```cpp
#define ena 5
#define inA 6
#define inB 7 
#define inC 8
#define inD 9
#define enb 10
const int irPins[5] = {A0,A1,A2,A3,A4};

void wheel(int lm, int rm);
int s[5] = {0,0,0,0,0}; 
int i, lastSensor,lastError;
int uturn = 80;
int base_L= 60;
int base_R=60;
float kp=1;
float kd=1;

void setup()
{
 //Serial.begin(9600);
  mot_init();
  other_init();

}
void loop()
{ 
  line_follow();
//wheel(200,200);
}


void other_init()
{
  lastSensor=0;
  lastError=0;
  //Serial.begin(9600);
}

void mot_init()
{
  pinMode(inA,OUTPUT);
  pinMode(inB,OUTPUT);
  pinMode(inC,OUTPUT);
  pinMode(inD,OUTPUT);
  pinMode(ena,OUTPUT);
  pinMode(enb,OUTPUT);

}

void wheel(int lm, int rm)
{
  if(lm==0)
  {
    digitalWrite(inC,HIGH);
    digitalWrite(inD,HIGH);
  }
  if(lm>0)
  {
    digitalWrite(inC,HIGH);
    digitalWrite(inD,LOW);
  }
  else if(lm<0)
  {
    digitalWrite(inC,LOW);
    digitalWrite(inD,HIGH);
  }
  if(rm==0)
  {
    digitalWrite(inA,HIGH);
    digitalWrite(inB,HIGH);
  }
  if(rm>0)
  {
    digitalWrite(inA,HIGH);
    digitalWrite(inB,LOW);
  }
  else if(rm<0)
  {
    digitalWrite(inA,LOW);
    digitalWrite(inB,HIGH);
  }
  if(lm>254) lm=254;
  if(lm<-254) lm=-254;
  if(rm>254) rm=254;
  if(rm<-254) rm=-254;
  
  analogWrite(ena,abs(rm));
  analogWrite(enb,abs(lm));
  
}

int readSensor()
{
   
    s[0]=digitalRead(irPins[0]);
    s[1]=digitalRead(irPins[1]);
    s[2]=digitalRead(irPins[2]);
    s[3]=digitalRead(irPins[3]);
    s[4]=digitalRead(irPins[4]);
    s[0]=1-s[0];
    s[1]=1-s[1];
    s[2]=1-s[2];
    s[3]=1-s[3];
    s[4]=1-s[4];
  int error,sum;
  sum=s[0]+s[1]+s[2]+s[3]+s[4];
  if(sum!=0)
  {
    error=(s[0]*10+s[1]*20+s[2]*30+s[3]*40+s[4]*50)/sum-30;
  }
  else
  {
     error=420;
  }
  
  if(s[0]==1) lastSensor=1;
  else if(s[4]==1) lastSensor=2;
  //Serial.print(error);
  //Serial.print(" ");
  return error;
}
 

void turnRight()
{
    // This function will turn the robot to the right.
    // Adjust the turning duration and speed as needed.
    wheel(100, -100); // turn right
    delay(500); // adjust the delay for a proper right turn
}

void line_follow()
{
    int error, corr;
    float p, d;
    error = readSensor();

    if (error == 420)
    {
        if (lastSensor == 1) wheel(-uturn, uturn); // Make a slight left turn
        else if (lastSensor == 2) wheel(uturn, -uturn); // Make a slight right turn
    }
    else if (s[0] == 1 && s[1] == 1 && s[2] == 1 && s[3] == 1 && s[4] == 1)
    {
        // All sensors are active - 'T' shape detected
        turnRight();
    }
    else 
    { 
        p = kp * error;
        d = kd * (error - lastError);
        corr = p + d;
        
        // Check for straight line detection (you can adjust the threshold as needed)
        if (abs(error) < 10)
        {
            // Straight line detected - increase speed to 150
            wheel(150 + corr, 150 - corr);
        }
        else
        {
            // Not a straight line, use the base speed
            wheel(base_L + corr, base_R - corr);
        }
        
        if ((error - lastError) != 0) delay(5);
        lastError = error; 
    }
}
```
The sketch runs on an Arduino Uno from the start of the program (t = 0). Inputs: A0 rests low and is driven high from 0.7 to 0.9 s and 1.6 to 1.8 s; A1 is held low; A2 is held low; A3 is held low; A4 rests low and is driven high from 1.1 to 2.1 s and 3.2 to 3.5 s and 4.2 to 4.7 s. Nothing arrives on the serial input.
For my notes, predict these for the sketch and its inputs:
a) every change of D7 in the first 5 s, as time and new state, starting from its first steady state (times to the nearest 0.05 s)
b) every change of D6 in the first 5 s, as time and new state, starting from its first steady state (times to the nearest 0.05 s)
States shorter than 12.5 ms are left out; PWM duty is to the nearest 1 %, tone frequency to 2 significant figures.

0 s high; 1.5 s low; 2.1 s high; 4.6 s low; 4.7 s high
0 s low; 1.5 s high; 2.1 s low; 4.6 s high; 4.7 s low
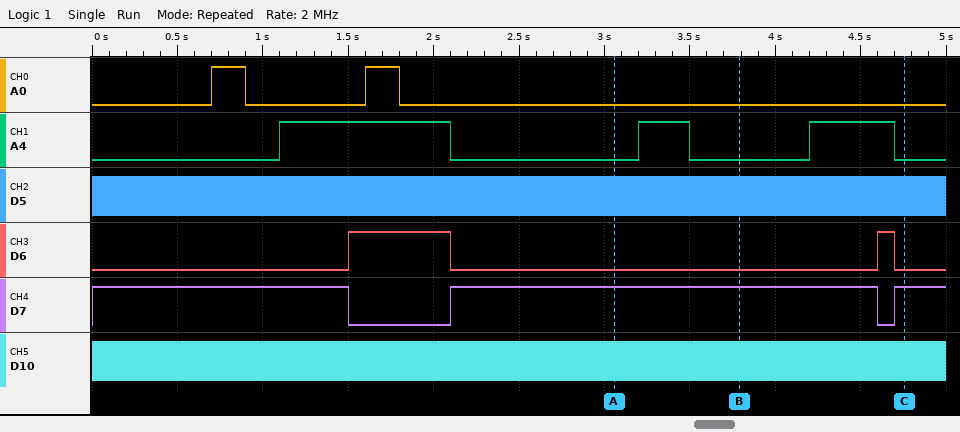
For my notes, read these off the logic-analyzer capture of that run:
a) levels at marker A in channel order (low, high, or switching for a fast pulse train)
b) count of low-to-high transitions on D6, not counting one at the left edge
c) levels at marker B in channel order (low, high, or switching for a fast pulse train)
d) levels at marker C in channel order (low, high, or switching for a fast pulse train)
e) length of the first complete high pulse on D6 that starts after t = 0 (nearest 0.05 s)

A0 low, A4 low, D5 switching, D6 low, D7 high, D10 switching
2
A0 low, A4 low, D5 switching, D6 low, D7 high, D10 switching
A0 low, A4 low, D5 switching, D6 low, D7 high, D10 switching
0.60 s
